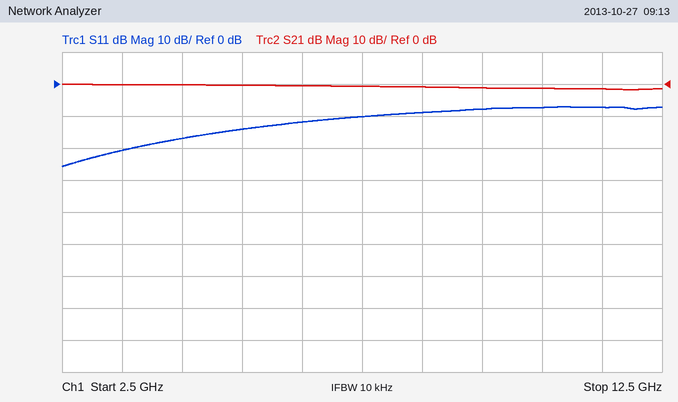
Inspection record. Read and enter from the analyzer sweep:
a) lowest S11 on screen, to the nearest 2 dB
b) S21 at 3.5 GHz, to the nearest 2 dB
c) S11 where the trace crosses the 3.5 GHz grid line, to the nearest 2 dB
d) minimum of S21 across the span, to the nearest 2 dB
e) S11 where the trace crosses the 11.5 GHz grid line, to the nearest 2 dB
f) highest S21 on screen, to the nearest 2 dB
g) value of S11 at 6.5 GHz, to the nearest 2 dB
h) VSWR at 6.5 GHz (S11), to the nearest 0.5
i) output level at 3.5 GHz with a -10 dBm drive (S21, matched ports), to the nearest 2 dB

-26 dB
0 dB
-20 dB
-2 dB
-8 dB
0 dB
-12 dB
1.5
-10 dBm
